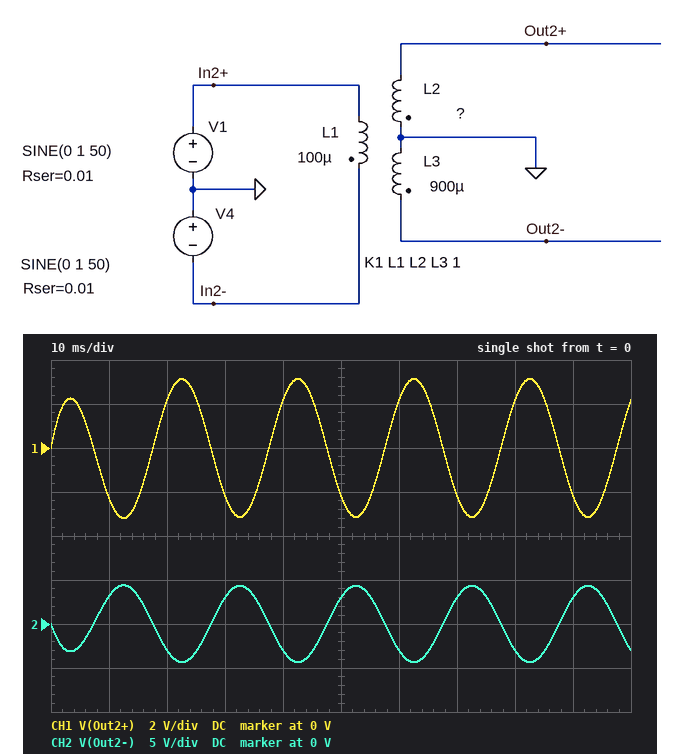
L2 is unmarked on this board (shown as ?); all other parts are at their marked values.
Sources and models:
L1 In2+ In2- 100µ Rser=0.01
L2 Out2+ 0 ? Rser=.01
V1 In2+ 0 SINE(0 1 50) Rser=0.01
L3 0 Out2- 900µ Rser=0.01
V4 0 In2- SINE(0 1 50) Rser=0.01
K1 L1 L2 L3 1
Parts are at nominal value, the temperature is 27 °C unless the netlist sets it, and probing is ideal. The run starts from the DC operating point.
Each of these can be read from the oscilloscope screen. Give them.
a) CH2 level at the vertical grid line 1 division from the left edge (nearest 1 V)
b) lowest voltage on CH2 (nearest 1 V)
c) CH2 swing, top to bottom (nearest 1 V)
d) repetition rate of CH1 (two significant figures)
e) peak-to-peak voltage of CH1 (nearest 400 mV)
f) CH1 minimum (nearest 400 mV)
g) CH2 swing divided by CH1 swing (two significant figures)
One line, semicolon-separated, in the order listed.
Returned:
3 V; -4 V; 9 V; 50 Hz; 6.4 V; -3.2 V; 1.4
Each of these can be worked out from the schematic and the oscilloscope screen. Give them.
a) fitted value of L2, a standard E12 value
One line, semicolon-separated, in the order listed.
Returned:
470 µH
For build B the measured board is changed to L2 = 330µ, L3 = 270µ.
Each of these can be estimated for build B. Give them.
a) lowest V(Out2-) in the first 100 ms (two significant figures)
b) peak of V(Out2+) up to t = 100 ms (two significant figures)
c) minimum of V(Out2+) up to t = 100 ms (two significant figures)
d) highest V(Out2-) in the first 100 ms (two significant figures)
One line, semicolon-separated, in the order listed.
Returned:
-2.4 V; 2.6 V; -2.7 V; 2.4 V
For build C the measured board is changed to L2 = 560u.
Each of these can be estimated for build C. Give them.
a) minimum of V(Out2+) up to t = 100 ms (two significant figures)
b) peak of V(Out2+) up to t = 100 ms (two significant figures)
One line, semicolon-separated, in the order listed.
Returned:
-3.5 V; 3.4 V
